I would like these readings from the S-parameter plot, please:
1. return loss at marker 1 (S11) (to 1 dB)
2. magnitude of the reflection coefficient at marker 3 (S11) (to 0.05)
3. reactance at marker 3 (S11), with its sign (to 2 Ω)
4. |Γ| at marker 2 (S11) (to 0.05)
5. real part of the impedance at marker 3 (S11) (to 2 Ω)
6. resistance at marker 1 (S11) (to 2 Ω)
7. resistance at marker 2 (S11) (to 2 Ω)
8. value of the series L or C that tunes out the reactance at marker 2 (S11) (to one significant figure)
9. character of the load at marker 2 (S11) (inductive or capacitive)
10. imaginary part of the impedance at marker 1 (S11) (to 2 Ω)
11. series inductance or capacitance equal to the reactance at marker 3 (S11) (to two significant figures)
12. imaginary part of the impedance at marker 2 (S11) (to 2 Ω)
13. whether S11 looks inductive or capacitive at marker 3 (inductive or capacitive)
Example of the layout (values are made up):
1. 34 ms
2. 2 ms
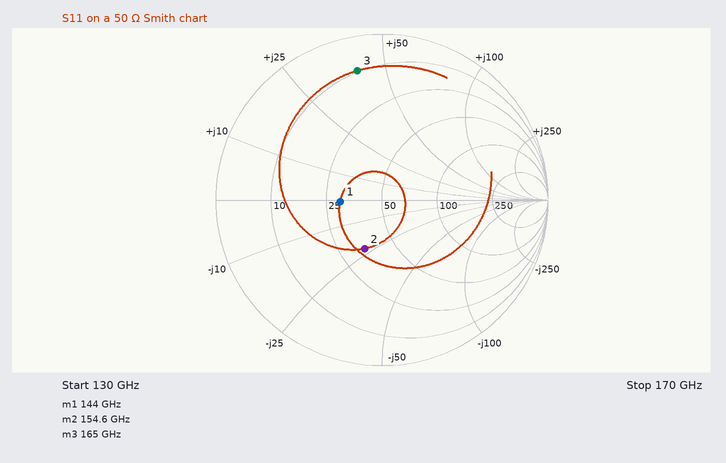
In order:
1. 12 dB
2. 0.80
3. +40 Ω
4. 0.30
5. 10 Ω
6. 30 Ω
7. 34 Ω
8. 20 pH
9. capacitive
10. 0 Ω
11. 39 pH
12. -22 Ω
13. inductive
